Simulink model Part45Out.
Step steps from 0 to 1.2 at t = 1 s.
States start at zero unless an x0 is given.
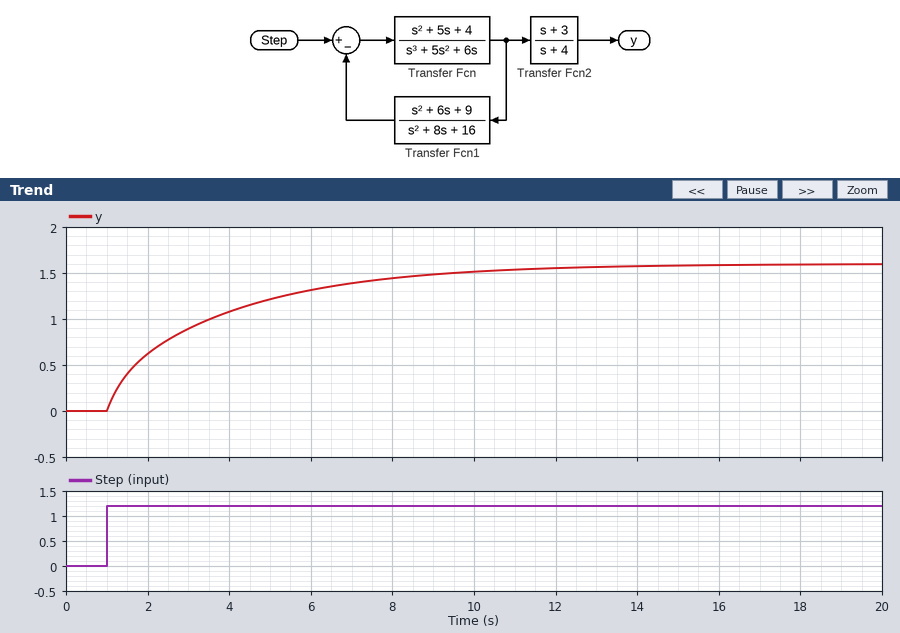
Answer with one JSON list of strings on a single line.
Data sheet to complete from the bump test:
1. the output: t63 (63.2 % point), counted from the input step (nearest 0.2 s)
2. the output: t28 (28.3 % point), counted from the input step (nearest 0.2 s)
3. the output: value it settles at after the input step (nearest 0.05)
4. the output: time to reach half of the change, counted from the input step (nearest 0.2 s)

["2.6 s", "0.6 s", "1.60", "1.6 s"]
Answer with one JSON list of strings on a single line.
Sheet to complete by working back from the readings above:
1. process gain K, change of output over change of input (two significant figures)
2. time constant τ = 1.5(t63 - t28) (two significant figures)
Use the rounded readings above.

["1.3", "3.0 s"]
